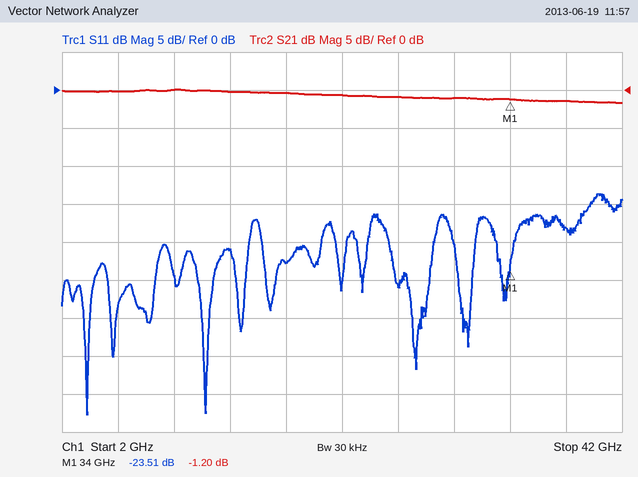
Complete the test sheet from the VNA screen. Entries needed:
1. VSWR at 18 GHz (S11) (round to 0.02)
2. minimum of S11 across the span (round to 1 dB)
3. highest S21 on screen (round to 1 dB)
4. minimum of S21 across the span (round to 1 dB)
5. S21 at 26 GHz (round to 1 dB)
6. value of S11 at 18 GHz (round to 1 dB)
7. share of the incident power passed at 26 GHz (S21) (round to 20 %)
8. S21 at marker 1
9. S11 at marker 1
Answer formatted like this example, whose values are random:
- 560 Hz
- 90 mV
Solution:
- 1.16
- -43 dB
- 0 dB
- -2 dB
- -1 dB
- -23 dB
- 80 %
- -1.20 dB
- -23.51 dB
